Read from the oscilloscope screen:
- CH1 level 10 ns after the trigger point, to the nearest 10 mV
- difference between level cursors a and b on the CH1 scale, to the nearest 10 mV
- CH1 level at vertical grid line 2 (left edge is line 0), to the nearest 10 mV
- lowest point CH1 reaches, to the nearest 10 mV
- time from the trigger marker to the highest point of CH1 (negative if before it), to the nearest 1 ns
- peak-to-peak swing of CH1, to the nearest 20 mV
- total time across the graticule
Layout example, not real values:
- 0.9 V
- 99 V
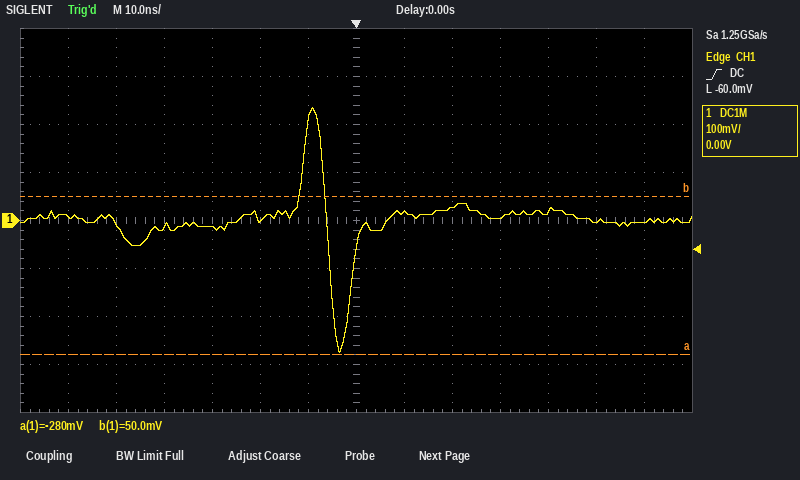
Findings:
- 20 mV
- 330 mV
- -10 mV
- -280 mV
- -9 ns
- 520 mV
- 140 ns
